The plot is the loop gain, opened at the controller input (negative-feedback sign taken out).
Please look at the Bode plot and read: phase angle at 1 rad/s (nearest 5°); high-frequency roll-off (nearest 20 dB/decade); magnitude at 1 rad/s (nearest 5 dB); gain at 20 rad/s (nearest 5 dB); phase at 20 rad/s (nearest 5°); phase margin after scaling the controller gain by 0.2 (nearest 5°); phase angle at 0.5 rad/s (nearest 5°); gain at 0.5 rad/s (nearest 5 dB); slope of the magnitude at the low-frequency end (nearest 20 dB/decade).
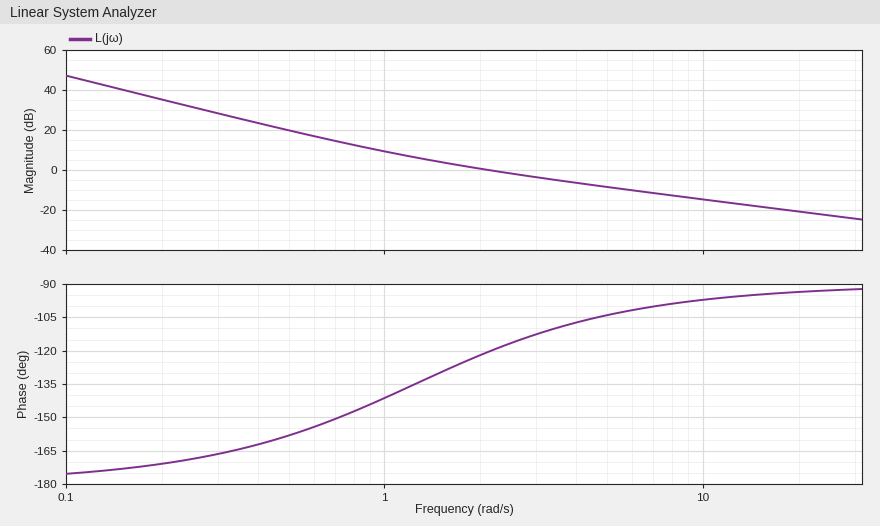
-140°
-20 dB/decade
10 dB
-20 dB
-95°
30°
-160°
20 dB
-40 dB/decade
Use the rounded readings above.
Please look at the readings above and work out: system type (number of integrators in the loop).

2
